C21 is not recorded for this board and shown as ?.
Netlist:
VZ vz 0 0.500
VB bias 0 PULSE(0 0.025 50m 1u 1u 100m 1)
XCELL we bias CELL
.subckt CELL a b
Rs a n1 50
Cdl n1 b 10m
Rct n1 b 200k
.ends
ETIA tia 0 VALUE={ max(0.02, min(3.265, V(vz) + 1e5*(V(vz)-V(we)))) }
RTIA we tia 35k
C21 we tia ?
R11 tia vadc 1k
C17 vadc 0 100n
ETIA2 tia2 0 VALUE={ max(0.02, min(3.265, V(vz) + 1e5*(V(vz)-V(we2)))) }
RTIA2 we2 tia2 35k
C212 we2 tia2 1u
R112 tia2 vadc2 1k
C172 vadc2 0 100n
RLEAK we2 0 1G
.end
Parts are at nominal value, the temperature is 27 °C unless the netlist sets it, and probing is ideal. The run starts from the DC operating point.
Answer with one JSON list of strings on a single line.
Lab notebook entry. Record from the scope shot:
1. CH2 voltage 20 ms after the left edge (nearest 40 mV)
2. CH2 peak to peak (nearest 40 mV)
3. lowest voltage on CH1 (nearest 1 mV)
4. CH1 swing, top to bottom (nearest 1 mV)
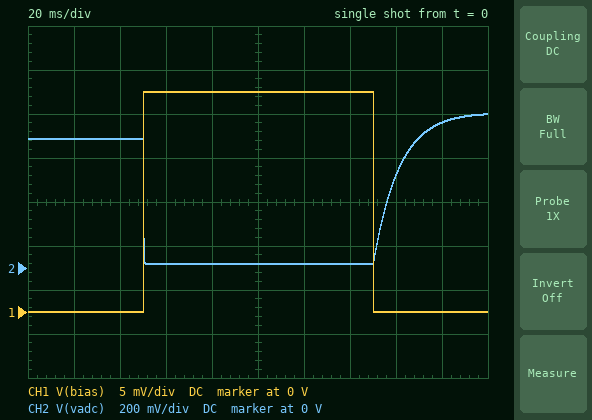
["600 mV", "680 mV", "0 V", "25 mV"]
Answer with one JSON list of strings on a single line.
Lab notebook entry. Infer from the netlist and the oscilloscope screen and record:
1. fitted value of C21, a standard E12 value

["330 nF"]
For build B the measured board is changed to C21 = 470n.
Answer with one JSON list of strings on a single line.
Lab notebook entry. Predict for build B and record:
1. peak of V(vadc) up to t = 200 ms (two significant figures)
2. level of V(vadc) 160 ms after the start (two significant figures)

["680 mV", "340 mV"]
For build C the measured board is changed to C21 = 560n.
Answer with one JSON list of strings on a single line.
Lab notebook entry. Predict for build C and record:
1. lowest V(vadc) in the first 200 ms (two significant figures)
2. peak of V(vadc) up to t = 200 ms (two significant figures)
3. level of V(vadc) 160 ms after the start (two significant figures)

["20 mV", "660 mV", "300 mV"]
